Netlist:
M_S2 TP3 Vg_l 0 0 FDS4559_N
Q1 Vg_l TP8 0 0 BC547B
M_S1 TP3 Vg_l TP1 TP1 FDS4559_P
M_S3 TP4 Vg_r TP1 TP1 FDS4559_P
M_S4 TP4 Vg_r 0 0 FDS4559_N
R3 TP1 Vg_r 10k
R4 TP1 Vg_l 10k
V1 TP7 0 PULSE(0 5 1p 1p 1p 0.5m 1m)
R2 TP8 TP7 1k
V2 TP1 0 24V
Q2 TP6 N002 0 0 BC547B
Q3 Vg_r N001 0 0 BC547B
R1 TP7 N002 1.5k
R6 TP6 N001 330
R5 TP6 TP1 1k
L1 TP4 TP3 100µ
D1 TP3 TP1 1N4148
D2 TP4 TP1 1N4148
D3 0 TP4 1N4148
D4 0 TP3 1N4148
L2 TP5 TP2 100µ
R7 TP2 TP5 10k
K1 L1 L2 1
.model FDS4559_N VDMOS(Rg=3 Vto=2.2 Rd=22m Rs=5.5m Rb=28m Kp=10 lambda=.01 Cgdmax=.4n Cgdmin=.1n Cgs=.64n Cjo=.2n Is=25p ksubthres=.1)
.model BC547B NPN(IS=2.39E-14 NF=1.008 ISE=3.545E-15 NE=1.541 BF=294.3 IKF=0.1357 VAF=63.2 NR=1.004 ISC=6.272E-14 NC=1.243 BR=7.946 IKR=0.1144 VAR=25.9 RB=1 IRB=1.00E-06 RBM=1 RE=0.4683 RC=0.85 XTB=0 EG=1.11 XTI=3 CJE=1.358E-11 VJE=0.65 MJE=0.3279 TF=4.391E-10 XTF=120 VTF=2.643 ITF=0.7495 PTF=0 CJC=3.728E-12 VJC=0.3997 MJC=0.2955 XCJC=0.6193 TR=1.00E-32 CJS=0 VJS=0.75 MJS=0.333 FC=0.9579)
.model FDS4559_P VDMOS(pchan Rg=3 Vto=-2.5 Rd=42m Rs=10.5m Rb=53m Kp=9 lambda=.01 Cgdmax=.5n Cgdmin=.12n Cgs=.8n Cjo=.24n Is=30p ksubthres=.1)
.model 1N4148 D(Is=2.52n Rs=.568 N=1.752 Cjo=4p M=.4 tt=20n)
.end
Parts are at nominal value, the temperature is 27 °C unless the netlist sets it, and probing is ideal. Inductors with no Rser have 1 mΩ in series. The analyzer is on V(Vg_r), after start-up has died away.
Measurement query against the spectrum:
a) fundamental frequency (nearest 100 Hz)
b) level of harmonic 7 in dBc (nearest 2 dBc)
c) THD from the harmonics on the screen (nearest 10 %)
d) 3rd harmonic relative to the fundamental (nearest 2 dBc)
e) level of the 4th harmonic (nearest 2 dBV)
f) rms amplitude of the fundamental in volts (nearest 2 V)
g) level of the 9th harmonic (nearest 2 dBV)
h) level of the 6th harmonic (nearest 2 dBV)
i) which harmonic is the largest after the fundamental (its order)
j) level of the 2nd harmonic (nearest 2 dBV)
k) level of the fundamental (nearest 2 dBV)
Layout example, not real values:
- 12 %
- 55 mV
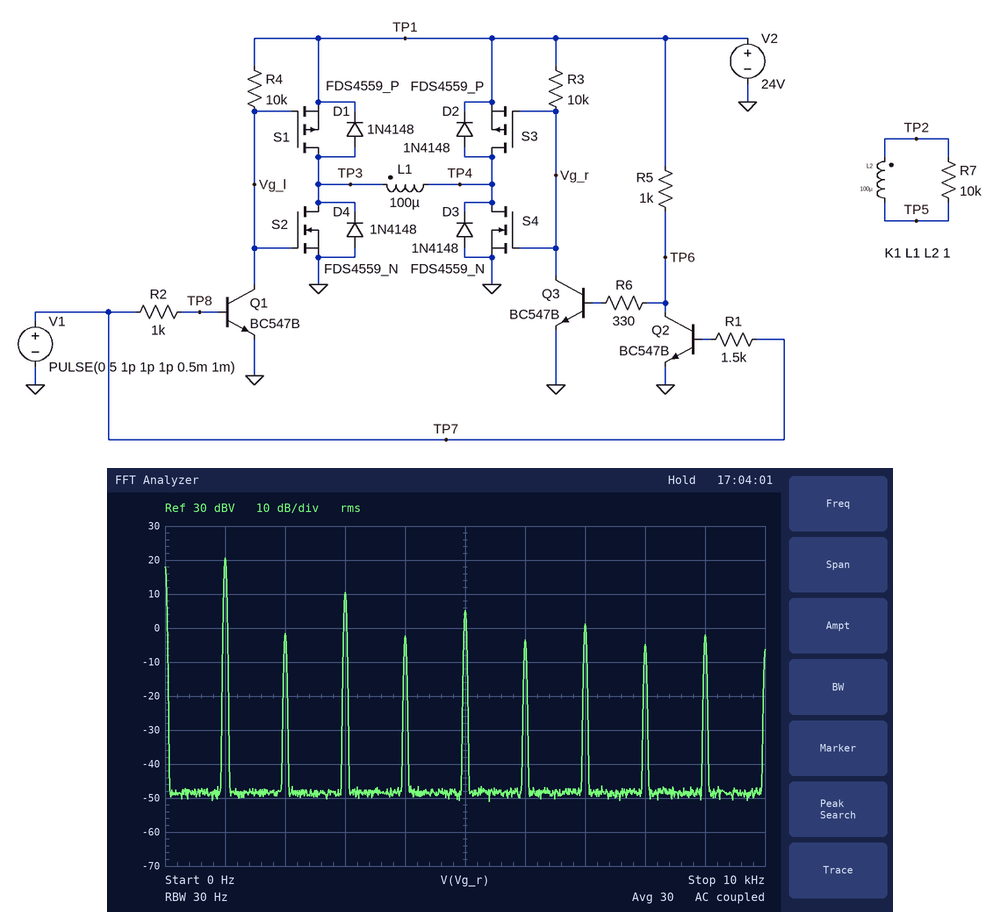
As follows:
- 1.0 kHz
- -20 dBc
- 40 %
- -10 dBc
- -2 dBV
- 10 V
- -2 dBV
- -4 dBV
- 3
- -2 dBV
- 20 dBV
